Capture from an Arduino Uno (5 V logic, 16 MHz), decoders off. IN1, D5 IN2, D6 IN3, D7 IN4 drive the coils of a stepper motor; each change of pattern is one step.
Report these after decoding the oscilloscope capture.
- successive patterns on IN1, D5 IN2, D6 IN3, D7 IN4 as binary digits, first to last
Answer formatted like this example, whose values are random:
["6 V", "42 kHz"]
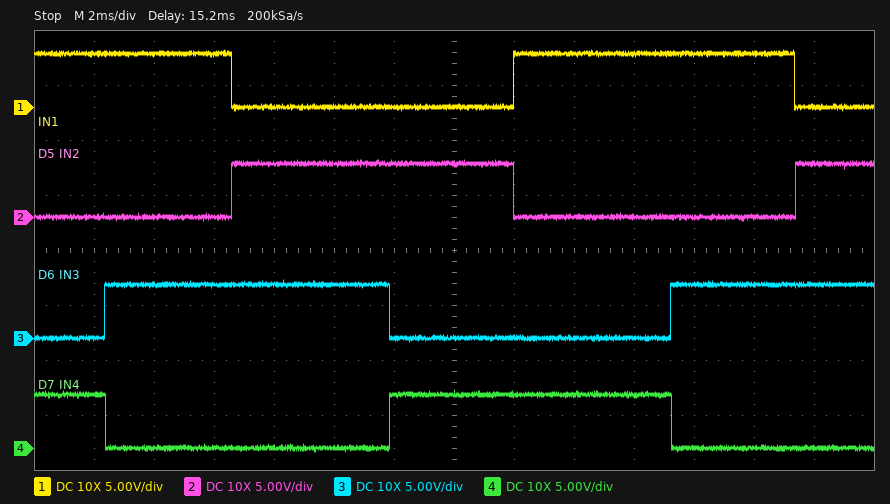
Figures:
["1001 1010 0110 0101 1001 1010 0110"]
